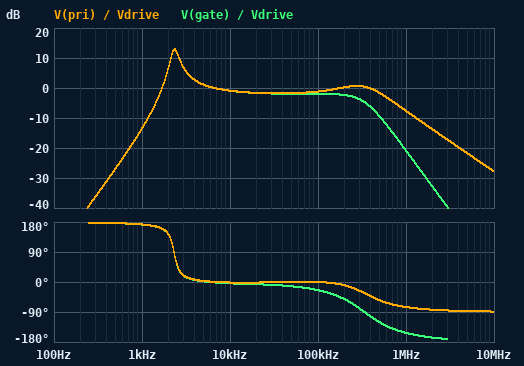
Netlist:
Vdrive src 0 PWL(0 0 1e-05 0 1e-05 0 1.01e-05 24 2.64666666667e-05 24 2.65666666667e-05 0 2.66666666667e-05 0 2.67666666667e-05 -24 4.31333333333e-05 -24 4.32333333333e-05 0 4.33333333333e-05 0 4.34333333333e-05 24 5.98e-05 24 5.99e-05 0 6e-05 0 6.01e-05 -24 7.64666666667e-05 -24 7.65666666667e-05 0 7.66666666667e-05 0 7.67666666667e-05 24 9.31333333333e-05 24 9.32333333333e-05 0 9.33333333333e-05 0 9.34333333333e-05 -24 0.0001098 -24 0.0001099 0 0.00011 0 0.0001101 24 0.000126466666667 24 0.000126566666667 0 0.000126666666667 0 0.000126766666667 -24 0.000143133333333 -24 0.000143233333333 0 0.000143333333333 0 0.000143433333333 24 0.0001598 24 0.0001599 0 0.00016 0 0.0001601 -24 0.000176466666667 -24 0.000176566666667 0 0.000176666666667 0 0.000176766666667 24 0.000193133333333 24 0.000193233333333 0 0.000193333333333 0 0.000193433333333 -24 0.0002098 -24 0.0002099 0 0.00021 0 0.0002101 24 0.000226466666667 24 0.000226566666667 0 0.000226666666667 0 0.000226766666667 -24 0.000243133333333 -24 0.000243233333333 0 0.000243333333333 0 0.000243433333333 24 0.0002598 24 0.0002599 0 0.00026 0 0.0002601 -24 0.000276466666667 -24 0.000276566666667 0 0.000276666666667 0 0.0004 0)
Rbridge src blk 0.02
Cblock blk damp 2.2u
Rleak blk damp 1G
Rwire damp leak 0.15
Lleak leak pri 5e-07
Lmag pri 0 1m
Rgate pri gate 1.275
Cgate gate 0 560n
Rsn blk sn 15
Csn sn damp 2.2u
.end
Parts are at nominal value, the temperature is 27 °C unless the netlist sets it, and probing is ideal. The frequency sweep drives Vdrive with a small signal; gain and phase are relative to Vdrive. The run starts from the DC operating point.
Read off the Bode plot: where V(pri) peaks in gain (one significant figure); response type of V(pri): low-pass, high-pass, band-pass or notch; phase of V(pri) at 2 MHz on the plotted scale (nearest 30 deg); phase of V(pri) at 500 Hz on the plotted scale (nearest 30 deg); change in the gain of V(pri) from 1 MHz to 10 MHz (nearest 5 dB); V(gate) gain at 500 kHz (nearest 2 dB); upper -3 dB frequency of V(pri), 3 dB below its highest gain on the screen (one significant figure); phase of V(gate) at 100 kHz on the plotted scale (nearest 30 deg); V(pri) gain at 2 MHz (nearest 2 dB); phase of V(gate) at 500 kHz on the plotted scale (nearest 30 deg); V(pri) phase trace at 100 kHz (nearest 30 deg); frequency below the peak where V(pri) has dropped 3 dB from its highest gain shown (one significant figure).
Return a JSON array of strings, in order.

["2 kHz", "band-pass", "-90 deg", "180 deg", "-20 dB", "-10 dB", "3 kHz", "-30 deg", "-14 dB", "-120 deg", "0 deg", "2 kHz"]
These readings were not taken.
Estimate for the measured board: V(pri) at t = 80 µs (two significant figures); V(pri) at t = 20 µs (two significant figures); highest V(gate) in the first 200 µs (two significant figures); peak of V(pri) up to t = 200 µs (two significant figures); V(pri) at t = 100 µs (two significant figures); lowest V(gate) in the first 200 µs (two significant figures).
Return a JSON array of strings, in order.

["16 V", "20 V", "20 V", "27 V", "-22 V", "-23 V"]
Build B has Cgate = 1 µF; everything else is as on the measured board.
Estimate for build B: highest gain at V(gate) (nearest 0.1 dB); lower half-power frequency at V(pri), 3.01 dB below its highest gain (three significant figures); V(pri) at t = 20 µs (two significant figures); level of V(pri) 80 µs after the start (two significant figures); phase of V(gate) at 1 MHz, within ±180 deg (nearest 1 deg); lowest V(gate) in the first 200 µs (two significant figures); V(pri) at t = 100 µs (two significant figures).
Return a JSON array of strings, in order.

["13.2 dB", "2.05 kHz", "17 V", "14 V", "-154 deg", "-20 V", "-19 V"]
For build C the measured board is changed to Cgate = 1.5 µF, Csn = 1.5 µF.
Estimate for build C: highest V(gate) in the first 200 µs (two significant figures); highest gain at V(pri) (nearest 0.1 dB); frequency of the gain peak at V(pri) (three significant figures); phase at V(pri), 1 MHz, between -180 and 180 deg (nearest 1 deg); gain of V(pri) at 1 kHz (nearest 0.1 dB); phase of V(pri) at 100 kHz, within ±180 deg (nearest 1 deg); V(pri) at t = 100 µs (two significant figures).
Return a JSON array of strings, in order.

["15 V", "17.1 dB", "2.23 kHz", "-69 deg", "-14.8 dB", "5 deg", "-16 V"]
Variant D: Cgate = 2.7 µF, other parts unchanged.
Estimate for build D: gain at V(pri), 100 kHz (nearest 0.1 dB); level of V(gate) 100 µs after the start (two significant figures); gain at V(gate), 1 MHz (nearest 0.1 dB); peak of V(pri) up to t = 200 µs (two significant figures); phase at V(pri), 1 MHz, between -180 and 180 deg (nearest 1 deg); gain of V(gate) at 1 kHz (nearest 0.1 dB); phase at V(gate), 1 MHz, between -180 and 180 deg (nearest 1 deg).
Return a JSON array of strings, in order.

["-2.1 dB", "-11 V", "-35.1 dB", "26 V", "-67 deg", "-12.5 dB", "-154 deg"]
